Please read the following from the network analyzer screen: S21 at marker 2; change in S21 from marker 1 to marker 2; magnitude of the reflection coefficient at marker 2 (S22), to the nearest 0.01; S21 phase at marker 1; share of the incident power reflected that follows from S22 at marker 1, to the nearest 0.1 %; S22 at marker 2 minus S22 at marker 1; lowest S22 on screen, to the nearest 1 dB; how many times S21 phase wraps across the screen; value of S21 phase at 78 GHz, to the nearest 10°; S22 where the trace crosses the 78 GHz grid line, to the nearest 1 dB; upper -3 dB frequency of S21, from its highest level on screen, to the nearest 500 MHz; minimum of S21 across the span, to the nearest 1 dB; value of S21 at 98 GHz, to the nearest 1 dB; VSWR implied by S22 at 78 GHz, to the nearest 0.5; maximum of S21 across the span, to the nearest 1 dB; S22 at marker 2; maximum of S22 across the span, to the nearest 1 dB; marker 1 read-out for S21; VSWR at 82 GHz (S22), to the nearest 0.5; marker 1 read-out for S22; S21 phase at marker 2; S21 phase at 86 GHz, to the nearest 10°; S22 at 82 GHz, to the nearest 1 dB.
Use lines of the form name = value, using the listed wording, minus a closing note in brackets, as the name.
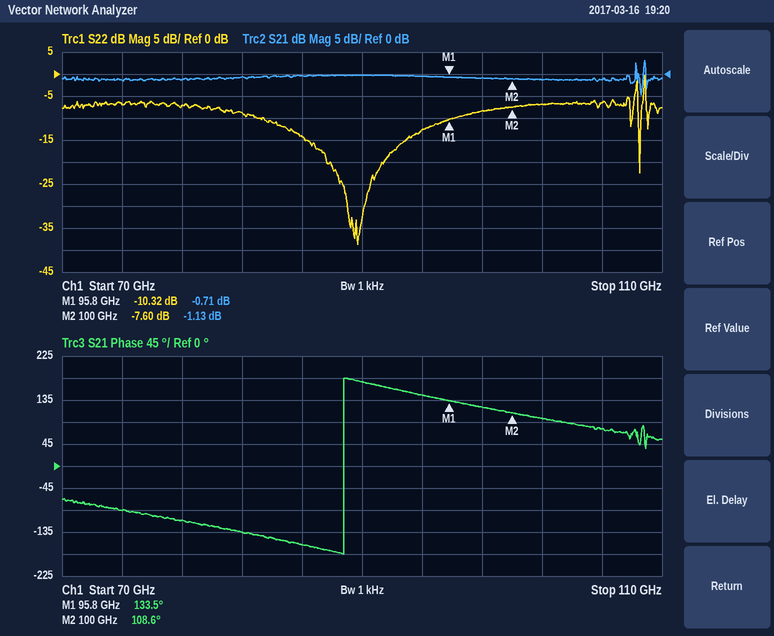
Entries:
S21 at marker 2 = -1.13 dB
change in S21 from marker 1 to marker 2 = -0.42 dB
magnitude of the reflection coefficient at marker 2 (S22), to the nearest 0.01 = 0.42
S21 phase at marker 1 = 133.5°
share of the incident power reflected that follows from S22 at marker 1, to the nearest 0.1 % = 9.3 %
S22 at marker 2 minus S22 at marker 1 = 2.72 dB
lowest S22 on screen, to the nearest 1 dB = -39 dB
how many times S21 phase wraps across the screen = 1
value of S21 phase at 78 GHz, to the nearest 10° = -110°
S22 where the trace crosses the 78 GHz grid line, to the nearest 1 dB = -7 dB
upper -3 dB frequency of S21, from its highest level on screen, to the nearest 500 MHz = 109.0 GHz
minimum of S21 across the span, to the nearest 1 dB = -5 dB
value of S21 at 98 GHz, to the nearest 1 dB = -1 dB
VSWR implied by S22 at 78 GHz, to the nearest 0.5 = 2.5
maximum of S21 across the span, to the nearest 1 dB = 3 dB
S22 at marker 2 = -7.60 dB
maximum of S22 across the span, to the nearest 1 dB = 0 dB
marker 1 read-out for S21 = -0.71 dB
VSWR at 82 GHz (S22), to the nearest 0.5 = 2.0
marker 1 read-out for S22 = -10.32 dB
S21 phase at marker 2 = 108.6°
S21 phase at 86 GHz, to the nearest 10° = -160°
S22 at 82 GHz, to the nearest 1 dB = -9 dB
